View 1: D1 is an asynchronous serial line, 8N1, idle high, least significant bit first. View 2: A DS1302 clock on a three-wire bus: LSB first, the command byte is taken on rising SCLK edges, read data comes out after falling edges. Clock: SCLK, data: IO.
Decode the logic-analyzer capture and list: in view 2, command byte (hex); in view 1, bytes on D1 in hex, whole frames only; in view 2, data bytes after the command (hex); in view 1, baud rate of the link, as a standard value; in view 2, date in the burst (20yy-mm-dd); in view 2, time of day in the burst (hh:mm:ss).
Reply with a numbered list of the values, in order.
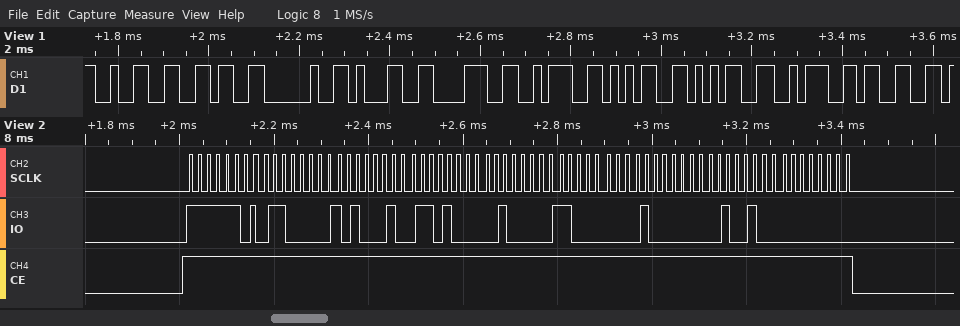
1. 0xBF
2. 32 36 20 31 38 3A 35 35 3A 33
3. 06 45 16 04 03 02 24 00
4. 57600 baud
5. 2024-03-04
6. 16:45:06
